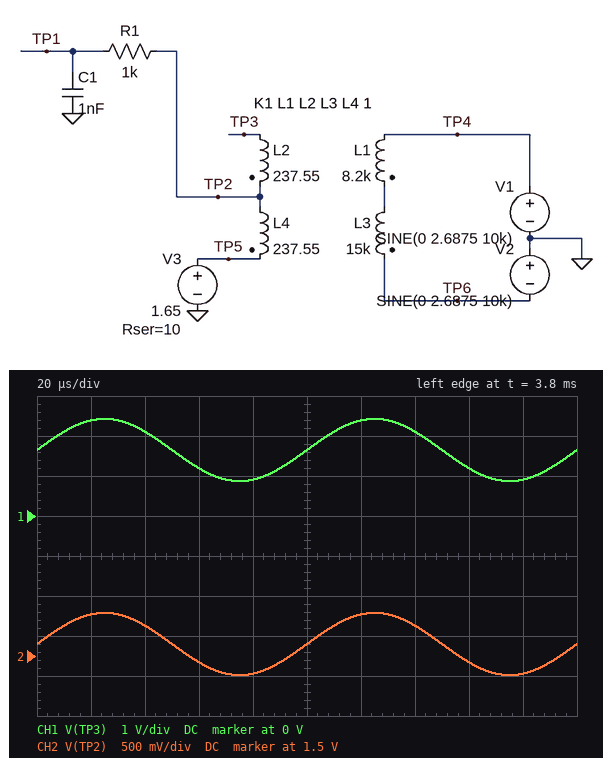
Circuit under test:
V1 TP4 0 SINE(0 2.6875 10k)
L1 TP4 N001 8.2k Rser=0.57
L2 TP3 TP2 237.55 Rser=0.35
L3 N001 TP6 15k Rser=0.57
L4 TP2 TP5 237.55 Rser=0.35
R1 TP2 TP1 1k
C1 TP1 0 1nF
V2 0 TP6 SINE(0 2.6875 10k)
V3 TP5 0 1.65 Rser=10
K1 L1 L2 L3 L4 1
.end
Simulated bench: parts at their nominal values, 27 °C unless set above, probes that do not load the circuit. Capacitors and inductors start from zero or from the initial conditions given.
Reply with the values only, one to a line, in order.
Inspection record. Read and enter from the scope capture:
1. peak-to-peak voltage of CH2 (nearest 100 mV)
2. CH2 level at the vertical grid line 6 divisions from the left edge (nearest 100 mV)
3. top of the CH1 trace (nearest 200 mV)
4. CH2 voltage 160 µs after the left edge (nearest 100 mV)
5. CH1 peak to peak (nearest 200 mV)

800 mV
2.0 V
2.4 V
1.4 V
1.6 V
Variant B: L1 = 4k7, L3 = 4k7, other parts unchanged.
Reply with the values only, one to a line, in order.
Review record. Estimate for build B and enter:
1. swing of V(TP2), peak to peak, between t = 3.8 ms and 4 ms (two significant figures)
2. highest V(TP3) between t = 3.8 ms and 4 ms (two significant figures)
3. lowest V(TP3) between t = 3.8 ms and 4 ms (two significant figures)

1.2 V
2.9 V
440 mV
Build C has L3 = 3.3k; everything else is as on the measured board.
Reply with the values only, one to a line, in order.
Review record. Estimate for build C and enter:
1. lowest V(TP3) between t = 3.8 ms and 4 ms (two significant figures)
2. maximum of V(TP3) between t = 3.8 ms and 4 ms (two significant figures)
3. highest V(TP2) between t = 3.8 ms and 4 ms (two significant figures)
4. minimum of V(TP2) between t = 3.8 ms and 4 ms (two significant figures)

530 mV
2.8 V
2.2 V
1.1 V
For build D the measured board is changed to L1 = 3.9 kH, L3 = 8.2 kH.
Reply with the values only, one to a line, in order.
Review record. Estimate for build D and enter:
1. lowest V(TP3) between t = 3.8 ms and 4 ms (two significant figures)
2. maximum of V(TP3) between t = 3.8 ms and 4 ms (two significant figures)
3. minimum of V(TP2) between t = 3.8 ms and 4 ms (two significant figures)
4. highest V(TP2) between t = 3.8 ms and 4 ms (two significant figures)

570 mV
2.7 V
1.1 V
2.2 V
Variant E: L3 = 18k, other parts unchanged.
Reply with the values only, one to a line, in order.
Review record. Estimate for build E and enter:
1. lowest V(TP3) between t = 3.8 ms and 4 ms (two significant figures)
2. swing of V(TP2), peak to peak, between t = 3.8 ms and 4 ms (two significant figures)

910 mV
740 mV
